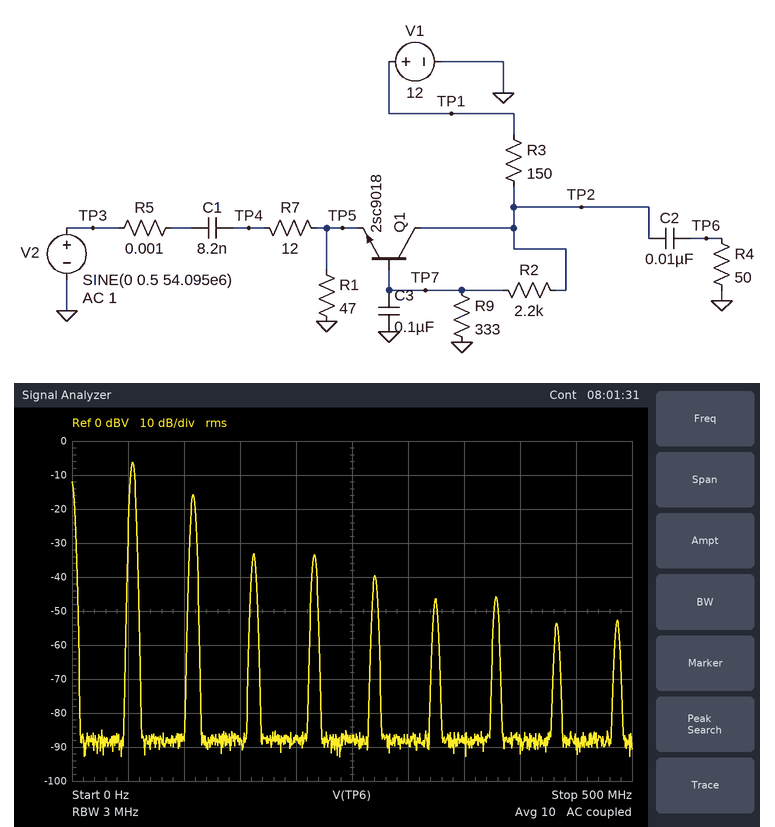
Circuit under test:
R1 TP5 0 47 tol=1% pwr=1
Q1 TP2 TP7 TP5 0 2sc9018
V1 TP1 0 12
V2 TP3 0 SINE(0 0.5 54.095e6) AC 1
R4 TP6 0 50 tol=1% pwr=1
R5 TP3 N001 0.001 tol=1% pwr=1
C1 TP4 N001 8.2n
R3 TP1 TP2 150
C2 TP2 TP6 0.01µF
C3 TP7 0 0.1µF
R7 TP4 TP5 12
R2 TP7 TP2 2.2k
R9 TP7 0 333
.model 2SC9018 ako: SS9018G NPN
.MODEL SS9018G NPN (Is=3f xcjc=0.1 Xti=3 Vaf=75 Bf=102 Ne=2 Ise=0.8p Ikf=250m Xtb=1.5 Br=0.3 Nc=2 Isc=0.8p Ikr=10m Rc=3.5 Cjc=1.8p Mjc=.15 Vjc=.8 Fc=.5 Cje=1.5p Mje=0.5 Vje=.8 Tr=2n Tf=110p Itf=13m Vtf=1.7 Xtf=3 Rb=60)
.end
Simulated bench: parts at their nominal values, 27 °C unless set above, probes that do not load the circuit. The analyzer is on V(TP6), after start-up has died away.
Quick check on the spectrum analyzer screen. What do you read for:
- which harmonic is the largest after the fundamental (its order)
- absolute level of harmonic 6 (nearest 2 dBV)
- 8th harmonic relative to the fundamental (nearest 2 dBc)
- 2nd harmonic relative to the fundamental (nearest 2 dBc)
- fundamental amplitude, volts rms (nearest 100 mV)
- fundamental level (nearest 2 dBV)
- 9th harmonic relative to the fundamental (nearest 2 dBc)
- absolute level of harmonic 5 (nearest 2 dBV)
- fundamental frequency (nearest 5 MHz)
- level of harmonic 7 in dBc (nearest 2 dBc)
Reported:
2
-46 dBV
-48 dBc
-10 dBc
500 mV
-6 dBV
-46 dBc
-40 dBV
55 MHz
-40 dBc
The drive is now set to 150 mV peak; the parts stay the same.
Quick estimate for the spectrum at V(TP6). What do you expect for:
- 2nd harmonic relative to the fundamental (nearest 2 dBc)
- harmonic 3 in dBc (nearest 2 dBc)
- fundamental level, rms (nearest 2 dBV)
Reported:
-26 dBc
-40 dBc
-12 dBV
